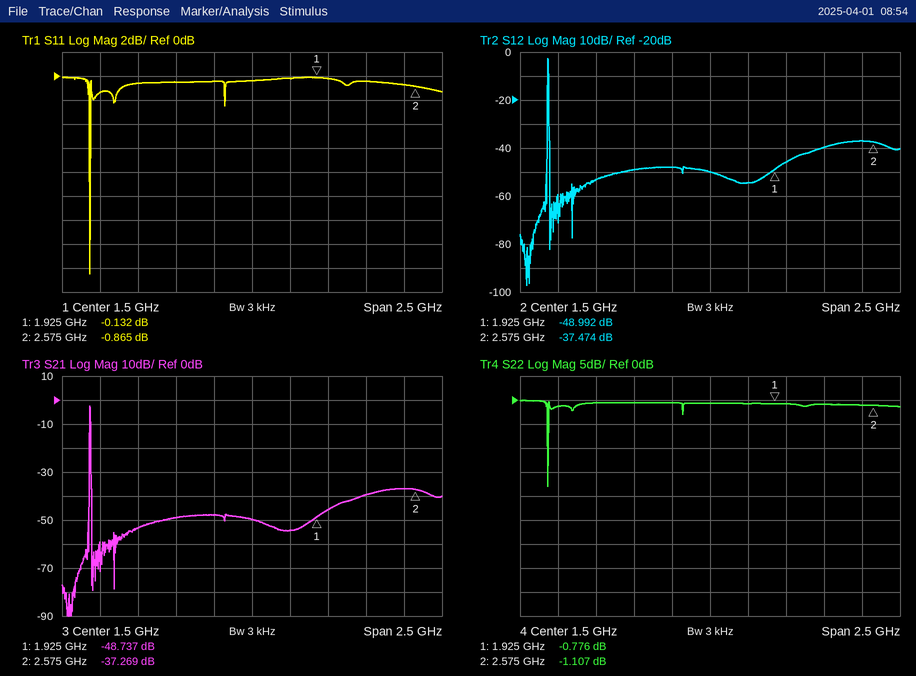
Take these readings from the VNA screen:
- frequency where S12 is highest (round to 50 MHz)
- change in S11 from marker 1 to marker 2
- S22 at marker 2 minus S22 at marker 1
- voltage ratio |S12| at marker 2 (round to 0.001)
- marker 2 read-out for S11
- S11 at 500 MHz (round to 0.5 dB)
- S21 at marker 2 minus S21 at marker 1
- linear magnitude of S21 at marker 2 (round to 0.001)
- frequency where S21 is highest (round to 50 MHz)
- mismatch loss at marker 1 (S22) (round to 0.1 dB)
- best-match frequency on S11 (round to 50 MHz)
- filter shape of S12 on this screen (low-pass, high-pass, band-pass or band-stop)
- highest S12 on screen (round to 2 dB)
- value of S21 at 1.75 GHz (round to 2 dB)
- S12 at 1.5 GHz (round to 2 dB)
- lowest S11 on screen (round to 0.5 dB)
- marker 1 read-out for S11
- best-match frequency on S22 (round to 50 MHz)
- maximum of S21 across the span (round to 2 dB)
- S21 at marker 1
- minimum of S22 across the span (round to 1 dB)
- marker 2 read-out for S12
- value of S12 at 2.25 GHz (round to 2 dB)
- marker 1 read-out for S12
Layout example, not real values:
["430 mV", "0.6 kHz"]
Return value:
["450 MHz", "-0.733 dB", "-0.331 dB", "0.013", "-0.865 dB", "-1.5 dB", "11.468 dB", "0.014", "450 MHz", "7.9 dB", "450 MHz", "band-pass", "-2 dB", "-54 dB", "-50 dB", "-16.5 dB", "-0.132 dB", "450 MHz", "-2 dB", "-48.737 dB", "-18 dB", "-37.474 dB", "-40 dB", "-48.992 dB"]
